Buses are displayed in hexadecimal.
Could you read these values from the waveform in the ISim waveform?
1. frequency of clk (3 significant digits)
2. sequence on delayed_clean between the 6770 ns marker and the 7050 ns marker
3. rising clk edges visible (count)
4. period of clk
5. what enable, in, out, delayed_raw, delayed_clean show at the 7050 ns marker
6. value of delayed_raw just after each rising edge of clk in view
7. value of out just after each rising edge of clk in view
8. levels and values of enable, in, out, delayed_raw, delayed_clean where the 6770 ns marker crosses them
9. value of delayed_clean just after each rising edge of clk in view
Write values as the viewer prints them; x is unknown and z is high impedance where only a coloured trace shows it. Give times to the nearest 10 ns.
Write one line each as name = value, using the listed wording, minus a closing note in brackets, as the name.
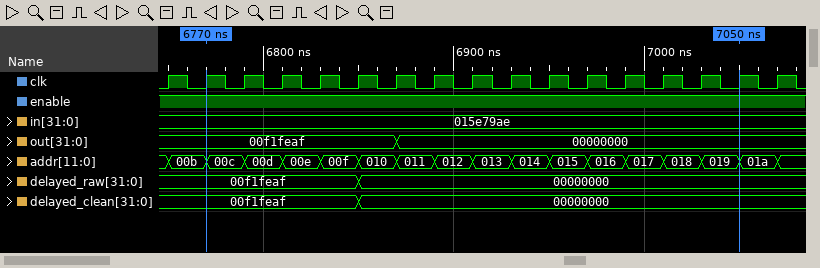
frequency of clk = 50.0 MHz
sequence on delayed_clean between the 6770 ns marker and the 7050 ns marker = 00f1feaf, 00000000
rising clk edges visible = 17
period of clk = 20 ns
what enable, in, out, delayed_raw, delayed_clean show at the 7050 ns marker = enable=1, in=015e79ae, out=00000000, delayed_raw=00000000, delayed_clean=00000000
value of delayed_raw just after each rising edge of clk in view = 00f1feaf, 00f1feaf, 00f1feaf, 00f1feaf, 00f1feaf, 00000000, 00000000, 00000000, 00000000, 00000000, 00000000, 00000000, 00000000, 00000000, 00000000, 00000000, 00000000
value of out just after each rising edge of clk in view = 00f1feaf, 00f1feaf, 00f1feaf, 00f1feaf, 00f1feaf, 00f1feaf, 00000000, 00000000, 00000000, 00000000, 00000000, 00000000, 00000000, 00000000, 00000000, 00000000, 00000000
levels and values of enable, in, out, delayed_raw, delayed_clean where the 6770 ns marker crosses them = enable=1, in=015e79ae, out=00f1feaf, delayed_raw=00f1feaf, delayed_clean=00f1feaf
value of delayed_clean just after each rising edge of clk in view = 00f1feaf, 00f1feaf, 00f1feaf, 00f1feaf, 00f1feaf, 00000000, 00000000, 00000000, 00000000, 00000000, 00000000, 00000000, 00000000, 00000000, 00000000, 00000000, 00000000
